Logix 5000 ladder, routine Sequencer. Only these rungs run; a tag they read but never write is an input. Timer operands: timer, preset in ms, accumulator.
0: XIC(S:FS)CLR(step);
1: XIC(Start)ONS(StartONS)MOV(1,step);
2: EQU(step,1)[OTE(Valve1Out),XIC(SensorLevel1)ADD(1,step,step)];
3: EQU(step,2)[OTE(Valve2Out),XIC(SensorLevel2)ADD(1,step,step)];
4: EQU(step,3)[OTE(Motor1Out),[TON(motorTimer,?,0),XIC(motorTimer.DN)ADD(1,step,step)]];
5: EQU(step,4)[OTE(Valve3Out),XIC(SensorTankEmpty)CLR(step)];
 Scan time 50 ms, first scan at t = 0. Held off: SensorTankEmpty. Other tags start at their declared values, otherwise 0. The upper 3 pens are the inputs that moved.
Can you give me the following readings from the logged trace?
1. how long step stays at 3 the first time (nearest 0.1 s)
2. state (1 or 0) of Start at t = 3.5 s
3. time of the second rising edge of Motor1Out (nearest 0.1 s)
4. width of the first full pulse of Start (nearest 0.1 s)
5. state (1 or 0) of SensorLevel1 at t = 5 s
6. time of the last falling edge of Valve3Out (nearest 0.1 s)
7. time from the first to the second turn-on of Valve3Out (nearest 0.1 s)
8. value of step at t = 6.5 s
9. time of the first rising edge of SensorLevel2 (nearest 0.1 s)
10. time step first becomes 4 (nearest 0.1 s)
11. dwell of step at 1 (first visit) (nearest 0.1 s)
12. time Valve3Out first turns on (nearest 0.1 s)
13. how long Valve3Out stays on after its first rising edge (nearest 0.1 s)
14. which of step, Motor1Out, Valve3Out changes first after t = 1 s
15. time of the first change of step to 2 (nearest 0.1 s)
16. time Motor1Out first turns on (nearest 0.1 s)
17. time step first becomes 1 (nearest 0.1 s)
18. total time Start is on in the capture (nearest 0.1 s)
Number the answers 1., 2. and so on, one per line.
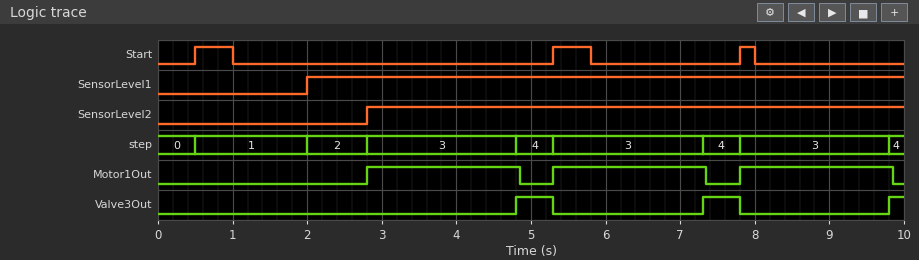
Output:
1. 2.0 s
2. 0
3. 5.3 s
4. 0.5 s
5. 1
6. 7.8 s
7. 2.5 s
8. 3
9. 2.8 s
10. 4.8 s
11. 1.5 s
12. 4.8 s
13. 0.5 s
14. step
15. 2.0 s
16. 2.8 s
17. 0.5 s
18. 1.2 s
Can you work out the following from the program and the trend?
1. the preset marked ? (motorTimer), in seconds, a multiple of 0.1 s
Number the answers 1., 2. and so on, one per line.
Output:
1. 2.0 s
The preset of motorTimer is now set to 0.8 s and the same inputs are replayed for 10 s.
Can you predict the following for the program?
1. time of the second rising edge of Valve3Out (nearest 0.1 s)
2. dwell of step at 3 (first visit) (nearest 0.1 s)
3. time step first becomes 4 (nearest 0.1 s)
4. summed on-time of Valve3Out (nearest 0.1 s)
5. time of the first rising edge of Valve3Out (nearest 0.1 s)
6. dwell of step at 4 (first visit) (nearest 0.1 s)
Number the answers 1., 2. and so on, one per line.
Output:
1. 6.1 s
2. 0.8 s
3. 3.6 s
4. 4.8 s
5. 3.6 s
6. 1.7 s
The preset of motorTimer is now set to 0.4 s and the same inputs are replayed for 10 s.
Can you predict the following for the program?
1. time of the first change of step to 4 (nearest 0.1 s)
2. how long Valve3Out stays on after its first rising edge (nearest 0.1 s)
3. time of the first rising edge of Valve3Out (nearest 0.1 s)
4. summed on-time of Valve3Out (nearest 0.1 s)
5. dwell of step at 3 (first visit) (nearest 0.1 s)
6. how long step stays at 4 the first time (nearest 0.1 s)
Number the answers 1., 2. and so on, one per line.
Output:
1. 3.2 s
2. 2.1 s
3. 3.2 s
4. 6.0 s
5. 0.4 s
6. 2.1 s
